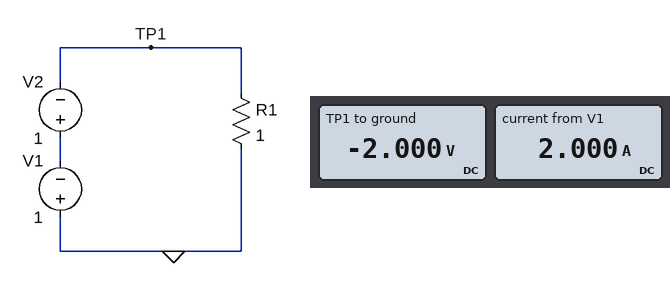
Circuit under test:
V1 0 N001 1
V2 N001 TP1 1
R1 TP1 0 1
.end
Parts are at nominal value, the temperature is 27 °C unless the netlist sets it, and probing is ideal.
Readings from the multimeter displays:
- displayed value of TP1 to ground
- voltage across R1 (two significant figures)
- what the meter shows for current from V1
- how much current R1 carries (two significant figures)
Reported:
-2.000 V
2.0 V
2.000 A
2.0 A
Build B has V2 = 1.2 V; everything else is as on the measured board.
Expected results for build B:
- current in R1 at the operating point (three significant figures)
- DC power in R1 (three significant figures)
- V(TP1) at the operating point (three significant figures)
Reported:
2.20 A
4.84 W
-2.20 V
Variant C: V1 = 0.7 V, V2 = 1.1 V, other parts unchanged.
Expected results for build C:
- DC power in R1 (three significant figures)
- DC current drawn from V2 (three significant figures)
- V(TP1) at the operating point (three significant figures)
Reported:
3.24 W
1.80 A
-1.80 V
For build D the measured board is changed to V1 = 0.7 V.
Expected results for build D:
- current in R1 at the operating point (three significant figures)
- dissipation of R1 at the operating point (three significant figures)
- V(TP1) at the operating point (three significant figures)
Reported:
1.70 A
2.89 W
-1.70 V
